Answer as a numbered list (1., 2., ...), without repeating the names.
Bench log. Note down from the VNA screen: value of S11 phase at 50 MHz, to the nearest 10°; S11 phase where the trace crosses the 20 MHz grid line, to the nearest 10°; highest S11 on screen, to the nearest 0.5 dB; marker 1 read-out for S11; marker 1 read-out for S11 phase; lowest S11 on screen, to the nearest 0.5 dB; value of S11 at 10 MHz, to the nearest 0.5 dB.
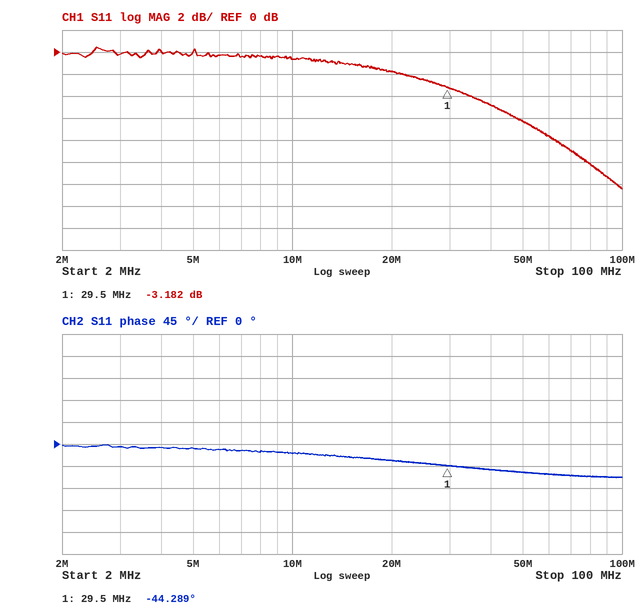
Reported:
1. -60°
2. -30°
3. 0.5 dB
4. -3.182 dB
5. -44.289°
6. -12.5 dB
7. -0.5 dB
